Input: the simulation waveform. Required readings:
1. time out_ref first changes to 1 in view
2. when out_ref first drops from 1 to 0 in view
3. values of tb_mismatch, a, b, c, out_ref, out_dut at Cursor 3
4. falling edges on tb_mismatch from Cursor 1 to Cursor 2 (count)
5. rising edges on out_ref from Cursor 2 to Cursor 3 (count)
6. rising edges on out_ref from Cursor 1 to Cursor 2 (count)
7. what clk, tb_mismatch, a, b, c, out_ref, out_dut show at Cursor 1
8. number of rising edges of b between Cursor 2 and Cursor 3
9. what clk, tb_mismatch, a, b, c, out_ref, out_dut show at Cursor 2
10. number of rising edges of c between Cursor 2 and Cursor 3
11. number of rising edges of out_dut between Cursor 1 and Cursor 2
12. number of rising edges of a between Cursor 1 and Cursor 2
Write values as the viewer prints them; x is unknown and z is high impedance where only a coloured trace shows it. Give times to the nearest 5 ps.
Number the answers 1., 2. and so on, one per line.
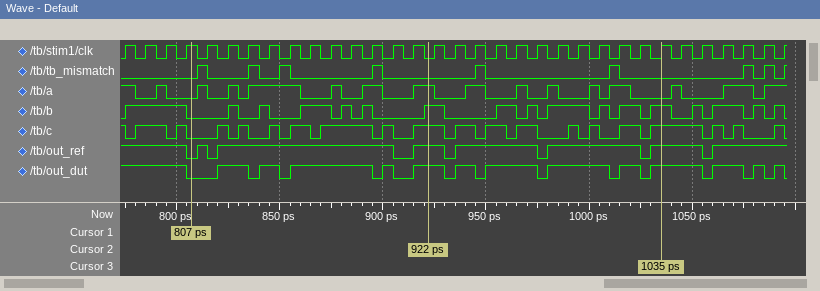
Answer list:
1. 810 ps
2. 805 ps
3. tb_mismatch=0, a=0, b=1, c=1, out_ref=1, out_dut=1
4. 4
5. 3
6. 3
7. clk=1, tb_mismatch=0, a=0, b=0, c=0, out_ref=0, out_dut=0
8. 6
9. clk=0, tb_mismatch=0, a=1, b=1, c=1, out_ref=1, out_dut=1
10. 7
11. 5
12. 6
